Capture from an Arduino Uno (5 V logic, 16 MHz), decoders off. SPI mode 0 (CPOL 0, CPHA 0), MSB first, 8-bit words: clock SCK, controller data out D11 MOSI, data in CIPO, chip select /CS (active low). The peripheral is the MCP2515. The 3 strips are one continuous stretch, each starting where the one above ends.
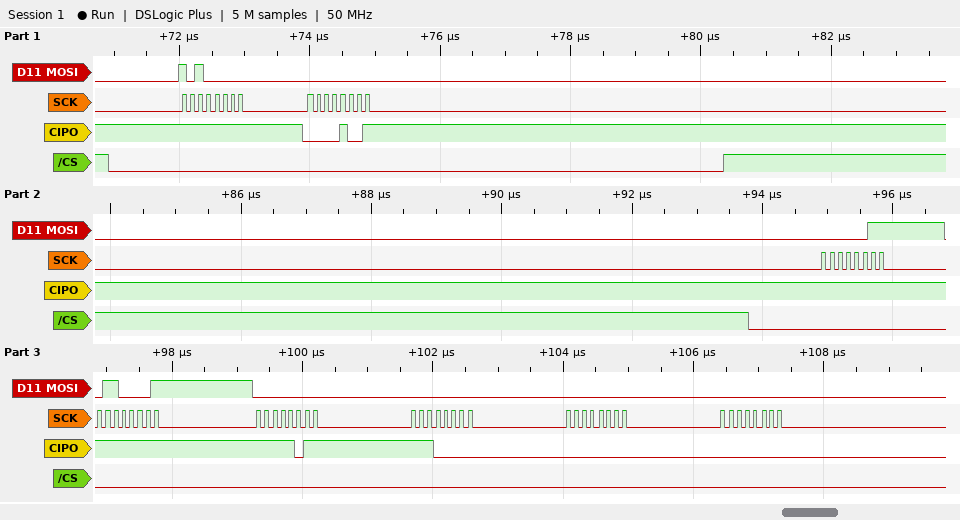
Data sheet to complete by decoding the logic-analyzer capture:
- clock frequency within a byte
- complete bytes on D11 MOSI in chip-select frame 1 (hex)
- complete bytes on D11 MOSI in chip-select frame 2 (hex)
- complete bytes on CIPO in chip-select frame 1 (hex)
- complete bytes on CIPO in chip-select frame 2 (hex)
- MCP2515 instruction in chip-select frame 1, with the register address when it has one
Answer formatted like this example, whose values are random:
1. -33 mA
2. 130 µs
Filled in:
1. 8 MHz
2. A0 00
3. 03 61 00 00 00 00
4. FF 09
5. FF FF FB E0 00 00
6. READ STATUS
